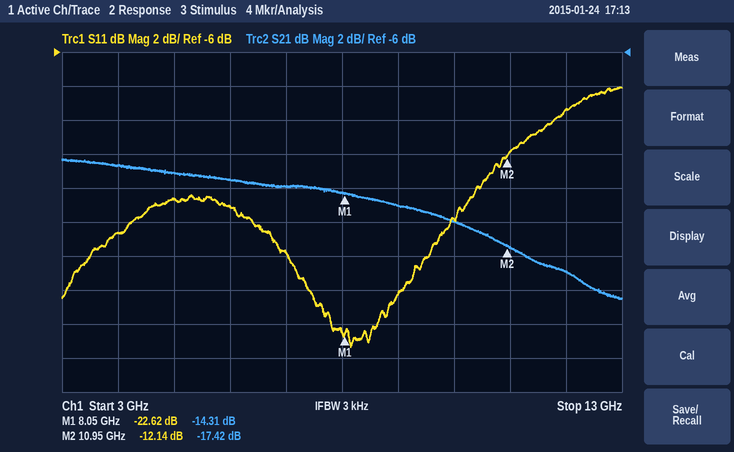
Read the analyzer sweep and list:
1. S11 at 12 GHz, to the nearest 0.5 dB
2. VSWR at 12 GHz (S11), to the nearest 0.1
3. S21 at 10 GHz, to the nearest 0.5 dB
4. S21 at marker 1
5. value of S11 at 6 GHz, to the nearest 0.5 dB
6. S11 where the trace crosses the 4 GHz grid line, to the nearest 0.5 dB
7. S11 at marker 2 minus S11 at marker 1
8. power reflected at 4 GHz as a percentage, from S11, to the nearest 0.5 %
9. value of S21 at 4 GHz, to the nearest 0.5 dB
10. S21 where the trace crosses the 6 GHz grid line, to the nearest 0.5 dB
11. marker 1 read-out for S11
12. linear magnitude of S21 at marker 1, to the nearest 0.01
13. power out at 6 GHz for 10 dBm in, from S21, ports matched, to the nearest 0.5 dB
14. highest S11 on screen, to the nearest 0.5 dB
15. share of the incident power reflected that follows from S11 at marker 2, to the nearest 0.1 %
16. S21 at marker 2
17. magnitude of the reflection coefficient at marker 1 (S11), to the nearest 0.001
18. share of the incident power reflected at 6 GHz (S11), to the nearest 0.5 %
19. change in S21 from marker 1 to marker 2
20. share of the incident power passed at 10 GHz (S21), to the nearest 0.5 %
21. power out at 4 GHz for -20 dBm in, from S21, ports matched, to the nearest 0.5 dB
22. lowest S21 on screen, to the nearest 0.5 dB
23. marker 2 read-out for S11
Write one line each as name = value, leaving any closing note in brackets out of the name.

S11 at 12 GHz, to the nearest 0.5 dB = -9.5 dB
VSWR at 12 GHz (S11), to the nearest 0.1 = 2.0
S21 at 10 GHz, to the nearest 0.5 dB = -16.0 dB
S21 at marker 1 = -14.31 dB
value of S11 at 6 GHz, to the nearest 0.5 dB = -15.0 dB
S11 where the trace crosses the 4 GHz grid line, to the nearest 0.5 dB = -16.5 dB
S11 at marker 2 minus S11 at marker 1 = 10.48 dB
power reflected at 4 GHz as a percentage, from S11, to the nearest 0.5 % = 2.0 %
value of S21 at 4 GHz, to the nearest 0.5 dB = -12.5 dB
S21 where the trace crosses the 6 GHz grid line, to the nearest 0.5 dB = -13.5 dB
marker 1 read-out for S11 = -22.62 dB
linear magnitude of S21 at marker 1, to the nearest 0.01 = 0.19
power out at 6 GHz for 10 dBm in, from S21, ports matched, to the nearest 0.5 dB = -3.5 dBm
highest S11 on screen, to the nearest 0.5 dB = -8.0 dB
share of the incident power reflected that follows from S11 at marker 2, to the nearest 0.1 % = 6.1 %
S21 at marker 2 = -17.42 dB
magnitude of the reflection coefficient at marker 1 (S11), to the nearest 0.001 = 0.074
share of the incident power reflected at 6 GHz (S11), to the nearest 0.5 % = 3.0 %
change in S21 from marker 1 to marker 2 = -3.11 dB
share of the incident power passed at 10 GHz (S21), to the nearest 0.5 % = 2.5 %
power out at 4 GHz for -20 dBm in, from S21, ports matched, to the nearest 0.5 dB = -32.5 dBm
lowest S21 on screen, to the nearest 0.5 dB = -20.5 dB
marker 2 read-out for S11 = -12.14 dB
